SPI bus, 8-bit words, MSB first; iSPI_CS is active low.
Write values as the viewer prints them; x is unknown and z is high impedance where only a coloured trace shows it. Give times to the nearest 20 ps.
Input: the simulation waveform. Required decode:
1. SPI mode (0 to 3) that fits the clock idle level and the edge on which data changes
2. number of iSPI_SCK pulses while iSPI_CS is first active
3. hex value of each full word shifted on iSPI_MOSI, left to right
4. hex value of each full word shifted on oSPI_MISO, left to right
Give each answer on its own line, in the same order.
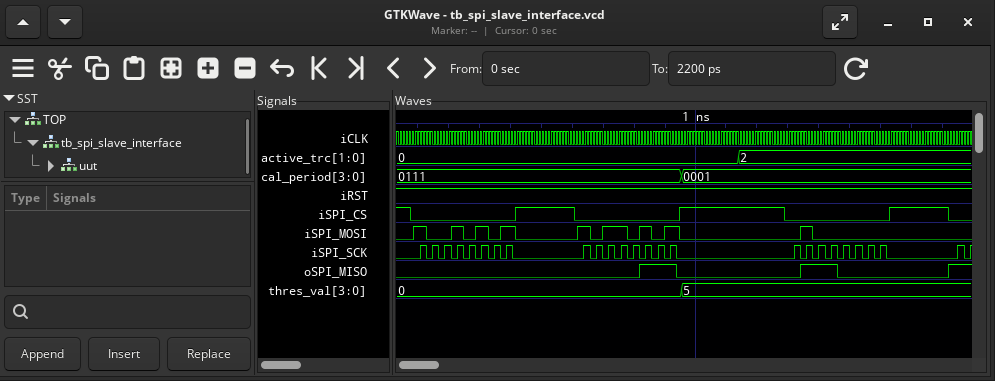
0
8
95, B5, 40
00, 07, 70
